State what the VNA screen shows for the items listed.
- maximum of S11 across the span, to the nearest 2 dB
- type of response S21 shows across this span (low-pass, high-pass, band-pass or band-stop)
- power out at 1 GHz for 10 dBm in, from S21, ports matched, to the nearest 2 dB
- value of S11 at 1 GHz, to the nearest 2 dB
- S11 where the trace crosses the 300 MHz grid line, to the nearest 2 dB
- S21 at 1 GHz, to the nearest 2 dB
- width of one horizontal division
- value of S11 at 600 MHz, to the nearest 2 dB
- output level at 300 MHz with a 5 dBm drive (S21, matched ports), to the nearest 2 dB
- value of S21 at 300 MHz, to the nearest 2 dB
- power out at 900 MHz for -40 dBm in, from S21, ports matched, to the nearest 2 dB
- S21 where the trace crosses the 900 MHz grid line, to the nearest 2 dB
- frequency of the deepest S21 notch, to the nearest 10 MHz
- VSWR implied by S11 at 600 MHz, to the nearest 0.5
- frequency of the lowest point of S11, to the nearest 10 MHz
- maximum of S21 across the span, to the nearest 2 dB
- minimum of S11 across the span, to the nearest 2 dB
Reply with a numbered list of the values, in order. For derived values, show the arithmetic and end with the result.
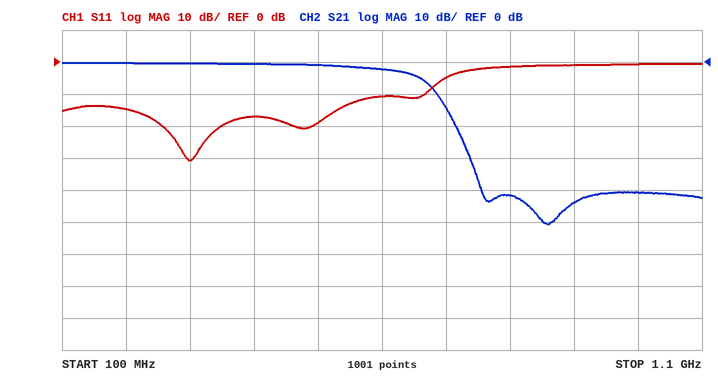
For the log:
1. 0 dB
2. low-pass
3. 10 dBm + (-40 dB) = -30 dBm
4. 0 dB
5. -30 dB
6. -40 dB
7. 100 MHz
8. -10 dB
9. 5 dBm + (0 dB) = 4 dBm
10. 0 dB
11. -40 dBm + (-44 dB) = -84 dBm
12. -44 dB
13. 860 MHz
14. |Γ| = 10^(-10/20) = 0.3162; VSWR = (1 + 0.3162)/(1 − 0.3162) ≈ 1.92, so 2.0 to the nearest 0.5
15. 300 MHz
16. 0 dB
17. -30 dB
